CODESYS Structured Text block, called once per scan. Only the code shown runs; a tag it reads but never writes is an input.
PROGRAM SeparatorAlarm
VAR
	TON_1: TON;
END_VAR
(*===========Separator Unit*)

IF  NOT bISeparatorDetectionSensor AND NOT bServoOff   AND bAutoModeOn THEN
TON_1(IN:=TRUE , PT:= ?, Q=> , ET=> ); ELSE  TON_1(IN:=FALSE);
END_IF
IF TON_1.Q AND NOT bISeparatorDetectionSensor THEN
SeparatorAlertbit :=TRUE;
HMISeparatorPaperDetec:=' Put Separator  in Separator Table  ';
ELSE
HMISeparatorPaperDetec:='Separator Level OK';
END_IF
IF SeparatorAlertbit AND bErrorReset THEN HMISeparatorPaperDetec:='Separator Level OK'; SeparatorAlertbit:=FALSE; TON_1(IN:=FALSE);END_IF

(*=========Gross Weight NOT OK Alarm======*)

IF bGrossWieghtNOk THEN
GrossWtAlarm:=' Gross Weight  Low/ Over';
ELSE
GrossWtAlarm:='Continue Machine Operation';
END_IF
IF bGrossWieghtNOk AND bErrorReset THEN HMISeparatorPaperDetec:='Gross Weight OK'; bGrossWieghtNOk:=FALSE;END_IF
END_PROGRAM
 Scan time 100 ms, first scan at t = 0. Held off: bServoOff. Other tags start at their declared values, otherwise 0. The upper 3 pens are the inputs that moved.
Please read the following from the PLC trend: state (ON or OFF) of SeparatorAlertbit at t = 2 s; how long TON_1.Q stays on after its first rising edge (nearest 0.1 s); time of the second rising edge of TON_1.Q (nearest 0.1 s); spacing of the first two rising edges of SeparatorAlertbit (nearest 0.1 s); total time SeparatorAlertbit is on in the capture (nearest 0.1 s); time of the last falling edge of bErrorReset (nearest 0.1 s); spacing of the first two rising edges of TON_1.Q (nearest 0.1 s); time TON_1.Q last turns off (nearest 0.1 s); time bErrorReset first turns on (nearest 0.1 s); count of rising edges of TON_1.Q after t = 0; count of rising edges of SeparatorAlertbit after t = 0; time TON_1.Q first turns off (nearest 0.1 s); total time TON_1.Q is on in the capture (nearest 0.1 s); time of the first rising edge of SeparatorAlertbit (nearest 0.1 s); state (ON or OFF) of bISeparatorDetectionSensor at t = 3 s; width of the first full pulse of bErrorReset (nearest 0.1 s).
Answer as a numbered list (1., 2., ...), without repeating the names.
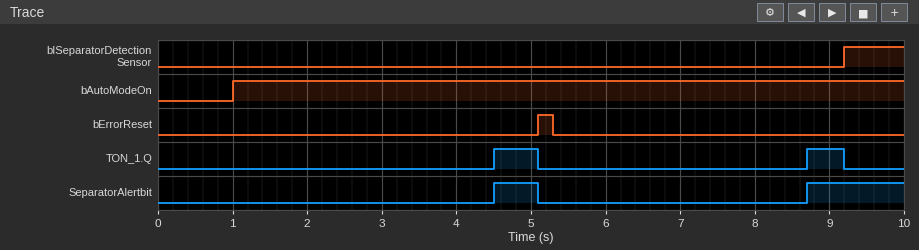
1. OFF
2. 0.6 s
3. 8.7 s
4. 4.2 s
5. 1.9 s
6. 5.3 s
7. 4.2 s
8. 9.2 s
9. 5.1 s
10. 2
11. 2
12. 5.1 s
13. 1.1 s
14. 4.5 s
15. OFF
16. 0.2 s
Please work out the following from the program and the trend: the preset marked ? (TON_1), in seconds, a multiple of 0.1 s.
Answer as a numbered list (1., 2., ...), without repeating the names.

1. 3.5 s
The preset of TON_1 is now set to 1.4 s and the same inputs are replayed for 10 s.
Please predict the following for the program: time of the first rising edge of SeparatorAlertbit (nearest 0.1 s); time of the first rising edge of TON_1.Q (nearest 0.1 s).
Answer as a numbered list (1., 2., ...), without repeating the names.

1. 2.4 s
2. 2.4 s
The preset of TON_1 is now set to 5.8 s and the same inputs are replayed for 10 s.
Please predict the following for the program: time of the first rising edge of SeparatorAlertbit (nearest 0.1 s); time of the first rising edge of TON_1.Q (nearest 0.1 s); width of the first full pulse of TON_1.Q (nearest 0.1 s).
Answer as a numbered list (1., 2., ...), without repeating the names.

1. 6.8 s
2. 6.8 s
3. 2.4 s
